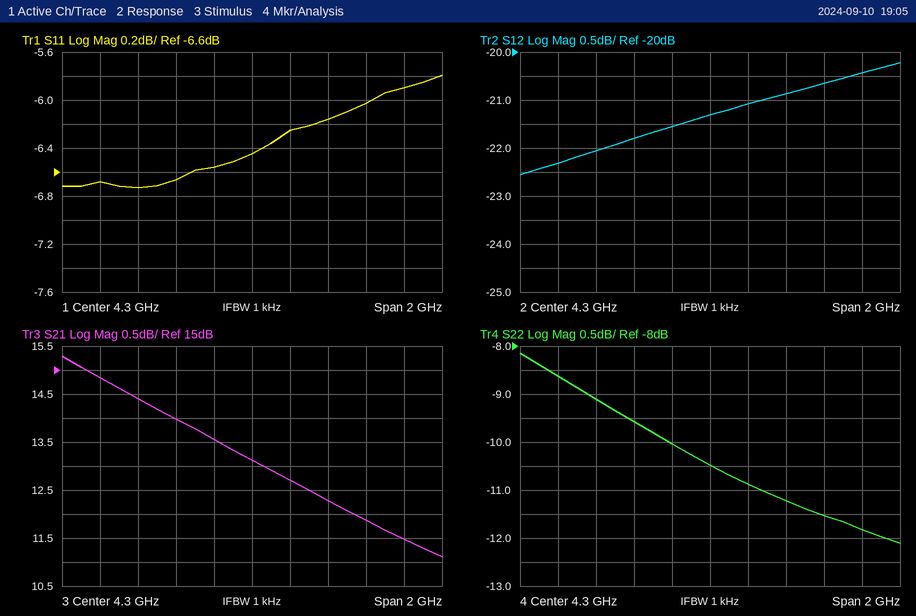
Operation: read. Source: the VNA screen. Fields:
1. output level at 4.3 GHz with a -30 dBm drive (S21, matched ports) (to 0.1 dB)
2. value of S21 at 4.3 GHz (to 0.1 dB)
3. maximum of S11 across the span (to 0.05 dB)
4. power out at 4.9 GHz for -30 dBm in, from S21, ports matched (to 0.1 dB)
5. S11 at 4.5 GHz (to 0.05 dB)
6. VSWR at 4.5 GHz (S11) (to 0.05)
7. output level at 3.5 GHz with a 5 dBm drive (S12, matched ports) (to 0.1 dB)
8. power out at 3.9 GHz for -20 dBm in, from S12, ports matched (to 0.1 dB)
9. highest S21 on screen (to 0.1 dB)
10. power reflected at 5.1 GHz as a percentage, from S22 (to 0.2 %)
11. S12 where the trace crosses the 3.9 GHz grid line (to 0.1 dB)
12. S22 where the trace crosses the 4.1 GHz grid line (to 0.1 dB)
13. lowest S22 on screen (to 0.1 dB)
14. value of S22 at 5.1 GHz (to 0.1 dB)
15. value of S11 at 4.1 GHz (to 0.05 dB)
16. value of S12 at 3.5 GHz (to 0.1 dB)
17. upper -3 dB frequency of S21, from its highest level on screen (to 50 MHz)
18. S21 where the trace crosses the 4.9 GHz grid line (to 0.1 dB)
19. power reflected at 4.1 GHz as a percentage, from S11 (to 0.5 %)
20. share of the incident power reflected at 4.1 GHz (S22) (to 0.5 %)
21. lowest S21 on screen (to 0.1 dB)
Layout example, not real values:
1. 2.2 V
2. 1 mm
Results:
1. -16.9 dBm
2. 13.1 dB
3. -5.80 dB
4. -18.1 dBm
5. -6.25 dB
6. 2.90
7. -17.3 dBm
8. -41.8 dBm
9. 15.3 dB
10. 6.6 %
11. -21.8 dB
12. -10.0 dB
13. -12.1 dB
14. -11.8 dB
15. -6.55 dB
16. -22.3 dB
17. 4.70 GHz
18. 11.9 dB
19. 22.0 %
20. 10.0 %
21. 11.1 dB
